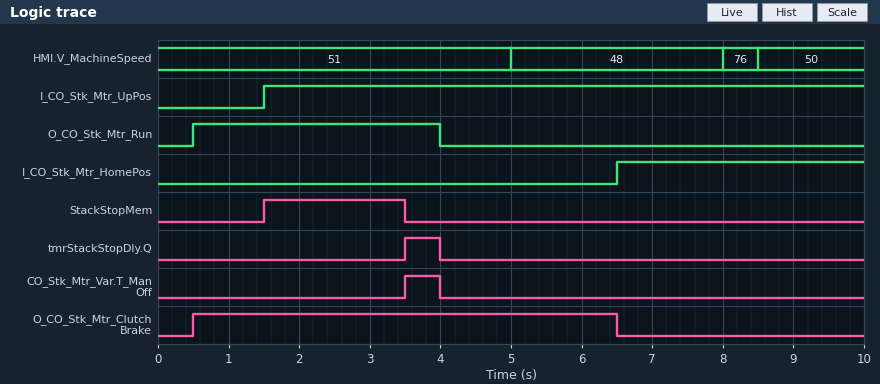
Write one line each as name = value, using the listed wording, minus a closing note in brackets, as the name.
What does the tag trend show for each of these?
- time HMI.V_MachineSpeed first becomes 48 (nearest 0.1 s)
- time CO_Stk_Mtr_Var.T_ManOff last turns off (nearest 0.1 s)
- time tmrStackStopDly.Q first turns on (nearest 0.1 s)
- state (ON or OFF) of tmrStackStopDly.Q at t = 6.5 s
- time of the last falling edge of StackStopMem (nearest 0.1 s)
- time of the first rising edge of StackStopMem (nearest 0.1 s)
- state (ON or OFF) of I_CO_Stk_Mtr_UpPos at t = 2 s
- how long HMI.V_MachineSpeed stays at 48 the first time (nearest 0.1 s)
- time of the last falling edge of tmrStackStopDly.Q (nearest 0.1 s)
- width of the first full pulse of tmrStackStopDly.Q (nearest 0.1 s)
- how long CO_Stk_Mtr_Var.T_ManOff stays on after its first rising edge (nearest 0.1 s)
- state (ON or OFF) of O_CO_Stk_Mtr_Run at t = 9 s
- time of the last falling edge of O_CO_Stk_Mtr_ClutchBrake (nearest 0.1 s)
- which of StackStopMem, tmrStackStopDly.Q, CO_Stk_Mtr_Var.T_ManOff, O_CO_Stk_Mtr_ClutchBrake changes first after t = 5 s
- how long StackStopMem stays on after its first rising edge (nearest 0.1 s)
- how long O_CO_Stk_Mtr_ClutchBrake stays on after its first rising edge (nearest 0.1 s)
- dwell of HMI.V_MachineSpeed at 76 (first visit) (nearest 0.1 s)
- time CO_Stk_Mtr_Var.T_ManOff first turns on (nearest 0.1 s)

time HMI.V_MachineSpeed first becomes 48 = 5.0 s
time CO_Stk_Mtr_Var.T_ManOff last turns off = 4.0 s
time tmrStackStopDly.Q first turns on = 3.5 s
state (ON or OFF) of tmrStackStopDly.Q at t = 6.5 s = OFF
time of the last falling edge of StackStopMem = 3.5 s
time of the first rising edge of StackStopMem = 1.5 s
state (ON or OFF) of I_CO_Stk_Mtr_UpPos at t = 2 s = ON
how long HMI.V_MachineSpeed stays at 48 the first time = 3.0 s
time of the last falling edge of tmrStackStopDly.Q = 4.0 s
width of the first full pulse of tmrStackStopDly.Q = 0.5 s
how long CO_Stk_Mtr_Var.T_ManOff stays on after its first rising edge = 0.5 s
state (ON or OFF) of O_CO_Stk_Mtr_Run at t = 9 s = OFF
time of the last falling edge of O_CO_Stk_Mtr_ClutchBrake = 6.5 s
which of StackStopMem, tmrStackStopDly.Q, CO_Stk_Mtr_Var.T_ManOff, O_CO_Stk_Mtr_ClutchBrake changes first after t = 5 s = O_CO_Stk_Mtr_ClutchBrake
how long StackStopMem stays on after its first rising edge = 2.0 s
how long O_CO_Stk_Mtr_ClutchBrake stays on after its first rising edge = 6.0 s
dwell of HMI.V_MachineSpeed at 76 (first visit) = 0.5 s
time CO_Stk_Mtr_Var.T_ManOff first turns on = 3.5 s
